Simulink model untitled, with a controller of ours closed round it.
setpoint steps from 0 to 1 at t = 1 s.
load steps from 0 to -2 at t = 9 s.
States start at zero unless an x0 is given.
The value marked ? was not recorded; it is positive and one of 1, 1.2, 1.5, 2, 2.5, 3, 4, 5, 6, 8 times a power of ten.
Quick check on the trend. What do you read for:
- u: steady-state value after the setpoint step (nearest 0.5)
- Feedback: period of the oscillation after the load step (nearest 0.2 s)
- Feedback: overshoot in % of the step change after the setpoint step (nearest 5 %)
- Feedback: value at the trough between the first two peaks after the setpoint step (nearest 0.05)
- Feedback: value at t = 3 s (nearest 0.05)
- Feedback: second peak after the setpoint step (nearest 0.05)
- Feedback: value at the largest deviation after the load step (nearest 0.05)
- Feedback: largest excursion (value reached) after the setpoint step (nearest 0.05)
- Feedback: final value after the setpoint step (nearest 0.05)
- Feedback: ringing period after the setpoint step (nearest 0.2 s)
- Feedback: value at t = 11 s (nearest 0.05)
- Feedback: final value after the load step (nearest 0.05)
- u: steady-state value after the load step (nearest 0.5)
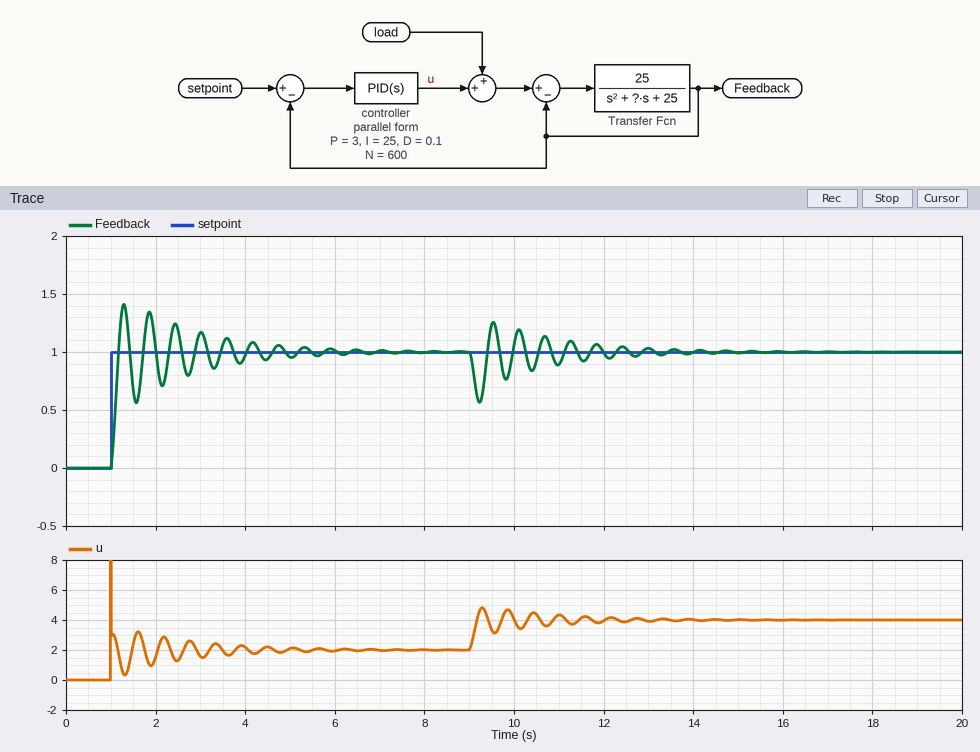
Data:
2.0
0.6 s
40 %
0.55
1.15
1.35
0.55
1.40
1.00
0.6 s
0.90
1.00
4.0
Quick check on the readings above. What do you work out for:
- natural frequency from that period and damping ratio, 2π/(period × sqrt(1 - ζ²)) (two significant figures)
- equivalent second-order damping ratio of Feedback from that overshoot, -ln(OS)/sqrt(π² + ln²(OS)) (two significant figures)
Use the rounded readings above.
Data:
11 rad/s
0.28
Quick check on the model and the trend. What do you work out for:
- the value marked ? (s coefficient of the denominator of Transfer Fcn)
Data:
4
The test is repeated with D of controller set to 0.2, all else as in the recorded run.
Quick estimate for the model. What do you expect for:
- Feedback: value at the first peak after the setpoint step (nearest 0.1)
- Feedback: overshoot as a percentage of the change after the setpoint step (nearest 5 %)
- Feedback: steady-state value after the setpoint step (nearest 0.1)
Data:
1.2
25 %
1.0
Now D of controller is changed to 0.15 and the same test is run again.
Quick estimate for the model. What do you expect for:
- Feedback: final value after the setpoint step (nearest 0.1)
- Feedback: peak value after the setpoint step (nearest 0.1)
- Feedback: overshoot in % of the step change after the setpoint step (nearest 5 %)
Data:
1.0
1.3
30 %
